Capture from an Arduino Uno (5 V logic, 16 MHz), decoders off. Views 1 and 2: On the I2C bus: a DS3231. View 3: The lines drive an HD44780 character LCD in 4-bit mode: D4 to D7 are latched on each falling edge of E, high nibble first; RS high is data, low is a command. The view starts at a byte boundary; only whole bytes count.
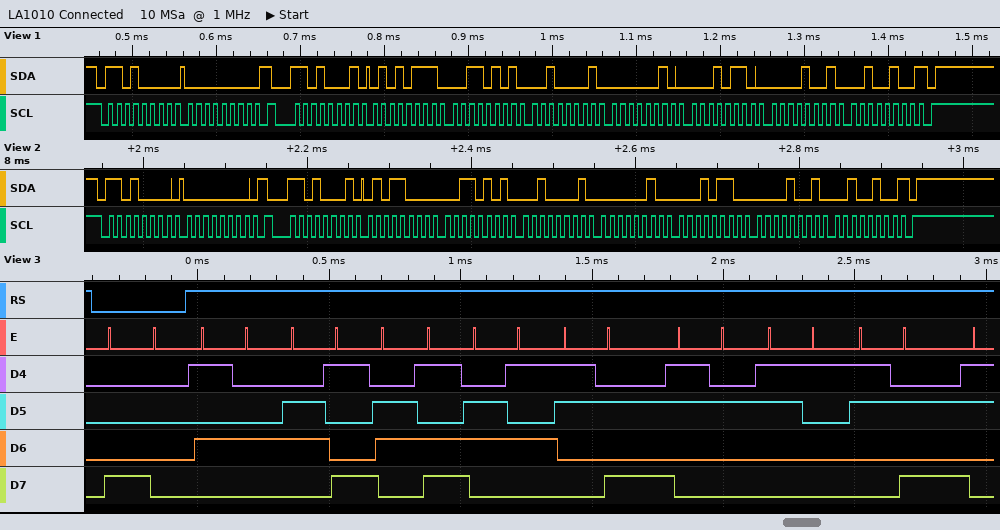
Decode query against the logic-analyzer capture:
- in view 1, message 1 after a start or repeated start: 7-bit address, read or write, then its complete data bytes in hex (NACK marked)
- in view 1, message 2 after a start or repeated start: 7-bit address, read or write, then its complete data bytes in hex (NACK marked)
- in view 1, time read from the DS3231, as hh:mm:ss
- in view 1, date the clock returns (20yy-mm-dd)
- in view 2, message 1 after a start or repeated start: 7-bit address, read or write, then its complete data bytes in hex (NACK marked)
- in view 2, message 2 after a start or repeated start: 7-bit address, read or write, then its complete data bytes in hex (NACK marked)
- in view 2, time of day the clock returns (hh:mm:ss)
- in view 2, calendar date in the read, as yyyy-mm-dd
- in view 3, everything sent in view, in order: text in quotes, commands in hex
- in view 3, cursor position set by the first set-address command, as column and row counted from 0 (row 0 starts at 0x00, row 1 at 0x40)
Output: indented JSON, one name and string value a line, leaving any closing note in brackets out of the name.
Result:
{
  "in view 1, message 1 after a start or repeated start: 7-bit address, read or write, then its complete data bytes in hex": "0x68 write: 00",
  "in view 1, message 2 after a start or repeated start: 7-bit address, read or write, then its complete data bytes in hex": "0x68 read: 57 35 21 02 16 09 24 NACK",
  "in view 1, time read from the DS3231, as hh:mm:ss": "21:35:57",
  "in view 1, date the clock returns": "2024-09-16",
  "in view 2, message 1 after a start or repeated start: 7-bit address, read or write, then its complete data bytes in hex": "0x68 write: 00",
  "in view 2, message 2 after a start or repeated start: 7-bit address, read or write, then its complete data bytes in hex": "0x68 read: 58 35 21 02 16 09 24 NACK",
  "in view 2, time of day the clock returns": "21:35:58",
  "in view 2, calendar date in the read, as yyyy-mm-dd": "2024-09-16",
  "in view 3, everything sent in view, in order: text in quotes, commands in hex": "0x80 \"Time:21:\"",
  "in view 3, cursor position set by the first set-address command, as column and row counted from 0": "column 0, row 0"
}
